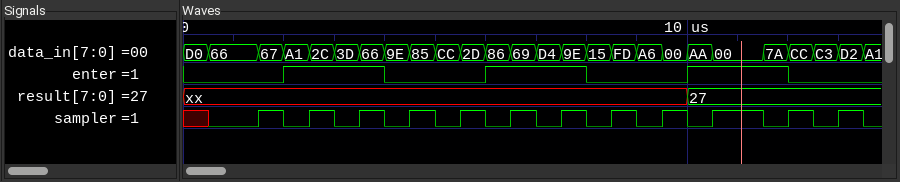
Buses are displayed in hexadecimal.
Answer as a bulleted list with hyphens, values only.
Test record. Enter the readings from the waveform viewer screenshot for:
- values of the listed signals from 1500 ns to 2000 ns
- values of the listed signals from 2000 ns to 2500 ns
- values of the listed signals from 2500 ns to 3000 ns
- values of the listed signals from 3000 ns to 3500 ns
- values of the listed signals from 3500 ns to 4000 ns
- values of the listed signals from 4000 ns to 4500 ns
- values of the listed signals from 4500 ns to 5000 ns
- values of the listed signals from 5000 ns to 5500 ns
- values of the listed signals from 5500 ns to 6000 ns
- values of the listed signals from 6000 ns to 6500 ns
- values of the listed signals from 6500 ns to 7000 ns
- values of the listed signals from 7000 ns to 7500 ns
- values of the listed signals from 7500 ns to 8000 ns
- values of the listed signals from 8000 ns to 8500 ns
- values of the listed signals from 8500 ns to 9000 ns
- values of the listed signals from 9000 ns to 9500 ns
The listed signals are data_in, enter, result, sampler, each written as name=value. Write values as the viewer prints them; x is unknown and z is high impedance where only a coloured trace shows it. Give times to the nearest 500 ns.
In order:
- data_in=67, enter=0, result=xx, sampler=1
- data_in=A1, enter=1, result=xx, sampler=0
- data_in=2C, enter=1, result=xx, sampler=1
- data_in=3D, enter=1, result=xx, sampler=0
- data_in=66, enter=1, result=xx, sampler=1
- data_in=9E, enter=0, result=xx, sampler=0
- data_in=85, enter=0, result=xx, sampler=1
- data_in=CC, enter=0, result=xx, sampler=0
- data_in=2D, enter=0, result=xx, sampler=1
- data_in=86, enter=1, result=xx, sampler=0
- data_in=69, enter=1, result=xx, sampler=1
- data_in=D4, enter=1, result=xx, sampler=0
- data_in=9E, enter=1, result=xx, sampler=1
- data_in=15, enter=0, result=xx, sampler=0
- data_in=FD, enter=0, result=xx, sampler=1
- data_in=A6, enter=0, result=xx, sampler=0
